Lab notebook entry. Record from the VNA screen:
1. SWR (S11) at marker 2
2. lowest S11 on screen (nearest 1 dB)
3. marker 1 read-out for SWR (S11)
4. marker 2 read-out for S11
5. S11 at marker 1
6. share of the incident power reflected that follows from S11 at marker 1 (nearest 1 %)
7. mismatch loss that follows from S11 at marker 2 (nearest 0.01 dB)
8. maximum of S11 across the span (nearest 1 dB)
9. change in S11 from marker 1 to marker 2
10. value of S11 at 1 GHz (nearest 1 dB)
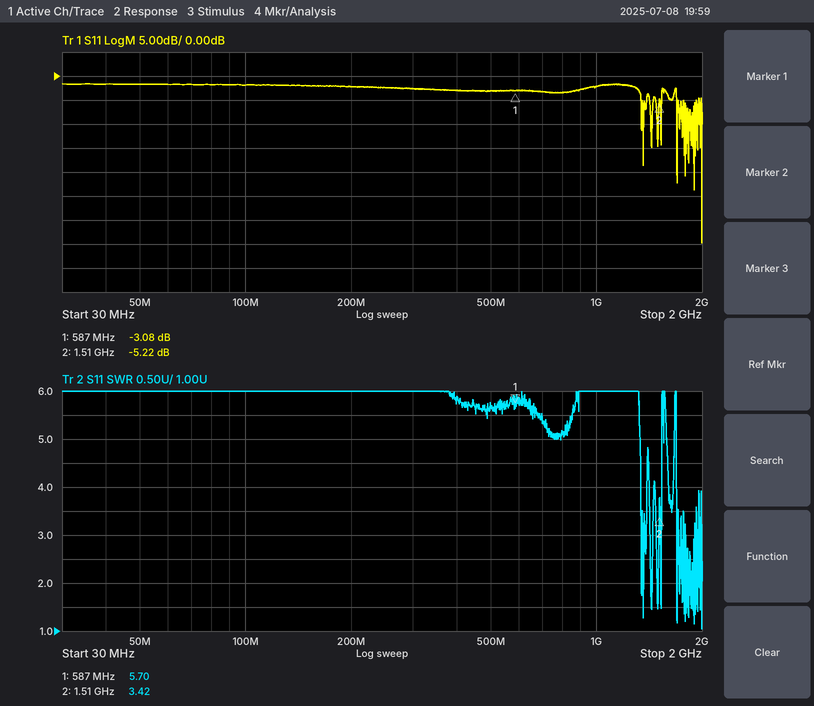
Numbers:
3.42
-35 dB
5.70
-5.22 dB
-3.08 dB
49 %
1.55 dB
-2 dB
-2.14 dB
-2 dB
